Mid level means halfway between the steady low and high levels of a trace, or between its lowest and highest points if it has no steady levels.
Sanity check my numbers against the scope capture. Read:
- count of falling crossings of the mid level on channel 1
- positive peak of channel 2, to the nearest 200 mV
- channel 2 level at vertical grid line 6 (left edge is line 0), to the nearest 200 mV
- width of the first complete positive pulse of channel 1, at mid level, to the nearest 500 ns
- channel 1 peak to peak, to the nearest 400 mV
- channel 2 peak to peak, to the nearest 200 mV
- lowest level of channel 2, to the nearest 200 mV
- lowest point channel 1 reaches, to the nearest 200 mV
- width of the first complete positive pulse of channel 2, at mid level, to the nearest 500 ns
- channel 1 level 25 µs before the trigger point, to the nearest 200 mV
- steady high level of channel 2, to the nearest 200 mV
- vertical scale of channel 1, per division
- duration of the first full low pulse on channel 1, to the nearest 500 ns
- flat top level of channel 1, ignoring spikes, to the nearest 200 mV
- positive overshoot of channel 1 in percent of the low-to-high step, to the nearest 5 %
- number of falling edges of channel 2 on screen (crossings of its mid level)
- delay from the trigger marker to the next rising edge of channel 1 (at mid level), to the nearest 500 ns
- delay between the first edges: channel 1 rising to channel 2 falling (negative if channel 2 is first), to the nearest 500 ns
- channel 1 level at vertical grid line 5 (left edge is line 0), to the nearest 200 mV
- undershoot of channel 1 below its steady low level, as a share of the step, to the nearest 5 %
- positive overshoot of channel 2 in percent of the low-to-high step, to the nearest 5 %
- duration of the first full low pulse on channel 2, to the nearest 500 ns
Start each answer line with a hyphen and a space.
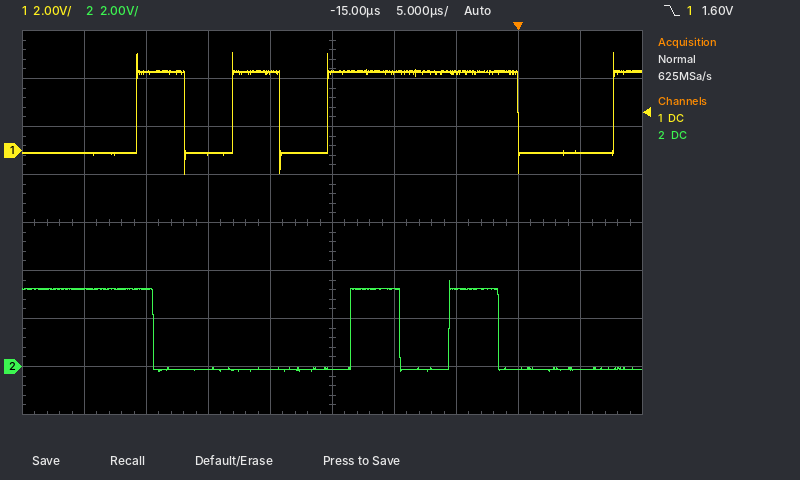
- 3
- 3.6 V
- 3.2 V
- 4.0 µs
- 5.2 V
- 3.8 V
- -200 mV
- -1.0 V
- 4.0 µs
- -200 mV
- 3.2 V
- 2 V
- 4.0 µs
- 3.2 V
- 25 %
- 3
- 7.5 µs
- +1.5 µs
- 3.2 V
- 25 %
- 10 %
- 16.0 µs
